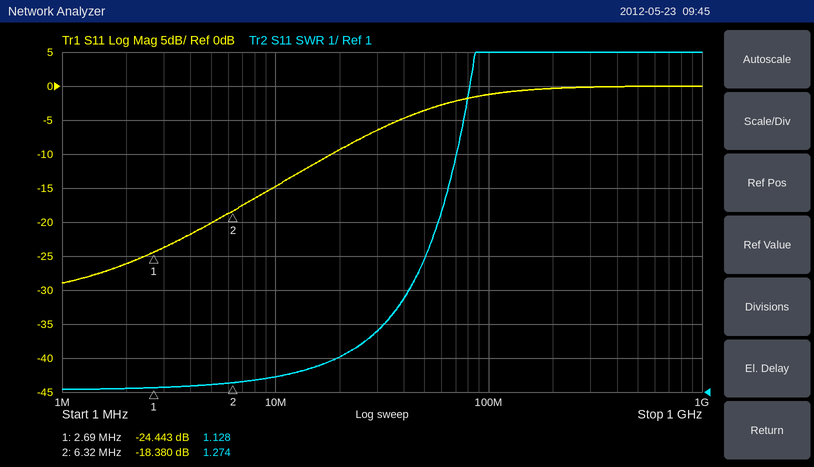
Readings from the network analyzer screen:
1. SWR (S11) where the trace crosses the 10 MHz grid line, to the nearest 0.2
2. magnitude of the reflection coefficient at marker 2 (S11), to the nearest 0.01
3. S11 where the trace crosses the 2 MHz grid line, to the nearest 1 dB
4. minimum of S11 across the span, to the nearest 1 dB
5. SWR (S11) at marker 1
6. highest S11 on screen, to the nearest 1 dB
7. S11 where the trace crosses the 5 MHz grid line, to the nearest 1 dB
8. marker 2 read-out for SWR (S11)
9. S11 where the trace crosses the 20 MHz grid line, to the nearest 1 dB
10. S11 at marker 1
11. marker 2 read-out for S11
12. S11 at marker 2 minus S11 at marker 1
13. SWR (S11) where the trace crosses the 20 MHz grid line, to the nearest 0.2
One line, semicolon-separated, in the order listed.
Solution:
1.4; 0.12; -26 dB; -29 dB; 1.128; 0 dB; -20 dB; 1.274; -9 dB; -24.443 dB; -18.380 dB; 6.063 dB; 2.0
